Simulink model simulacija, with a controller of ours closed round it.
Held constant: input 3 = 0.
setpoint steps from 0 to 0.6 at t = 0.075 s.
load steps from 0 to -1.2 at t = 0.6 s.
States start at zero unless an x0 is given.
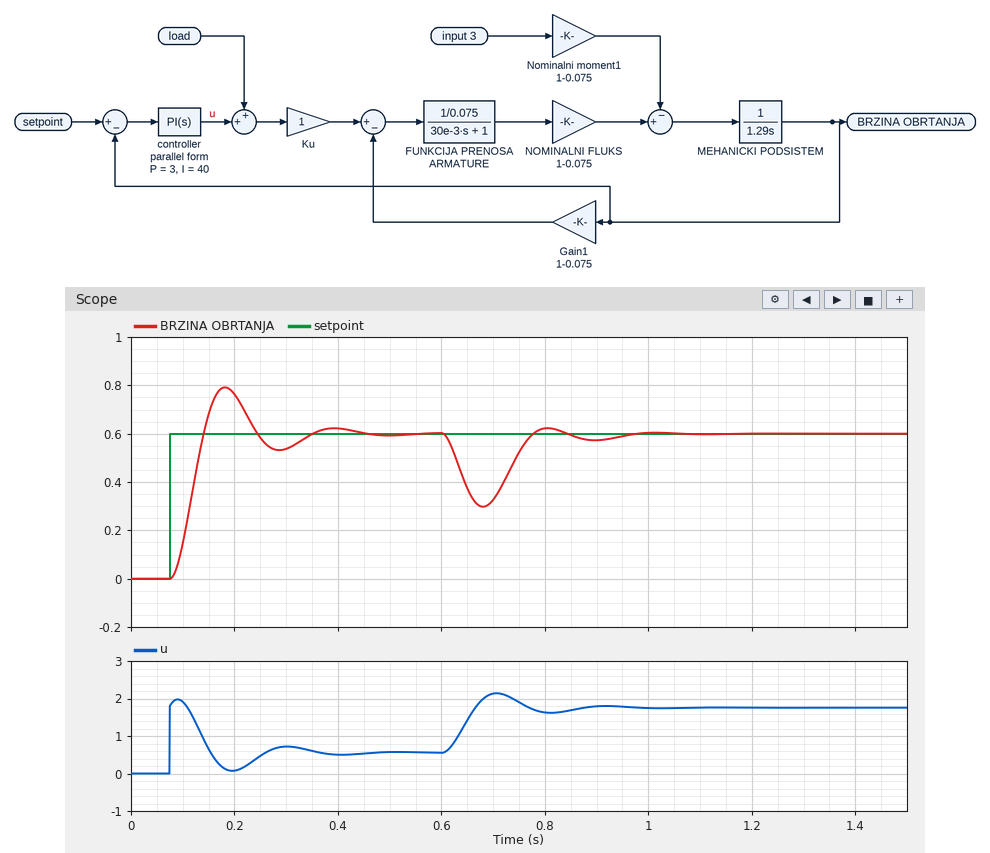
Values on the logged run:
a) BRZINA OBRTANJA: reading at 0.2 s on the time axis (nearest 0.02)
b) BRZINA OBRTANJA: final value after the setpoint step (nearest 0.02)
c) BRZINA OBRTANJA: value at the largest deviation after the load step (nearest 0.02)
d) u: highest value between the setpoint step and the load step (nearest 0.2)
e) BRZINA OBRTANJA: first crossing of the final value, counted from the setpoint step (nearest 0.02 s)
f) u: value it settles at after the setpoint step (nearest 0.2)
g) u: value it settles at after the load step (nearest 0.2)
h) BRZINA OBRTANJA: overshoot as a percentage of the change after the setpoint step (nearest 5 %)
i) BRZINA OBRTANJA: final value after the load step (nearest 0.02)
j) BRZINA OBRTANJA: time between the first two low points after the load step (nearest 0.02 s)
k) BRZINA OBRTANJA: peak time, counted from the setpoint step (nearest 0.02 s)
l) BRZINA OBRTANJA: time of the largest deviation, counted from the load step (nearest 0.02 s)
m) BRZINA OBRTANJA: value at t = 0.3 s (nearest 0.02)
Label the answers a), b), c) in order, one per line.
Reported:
a) 0.76
b) 0.60
c) 0.30
d) 2.0
e) 0.06 s
f) 0.6
g) 1.8
h) 30 %
i) 0.60
j) 0.22 s
k) 0.10 s
l) 0.08 s
m) 0.54
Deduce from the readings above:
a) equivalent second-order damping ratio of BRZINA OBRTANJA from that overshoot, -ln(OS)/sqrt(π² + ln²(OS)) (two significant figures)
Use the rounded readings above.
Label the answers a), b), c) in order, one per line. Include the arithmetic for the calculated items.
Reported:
a) ln(0.3) = -1.204; 1.204 / sqrt(9.870 + 1.450) = 0.36
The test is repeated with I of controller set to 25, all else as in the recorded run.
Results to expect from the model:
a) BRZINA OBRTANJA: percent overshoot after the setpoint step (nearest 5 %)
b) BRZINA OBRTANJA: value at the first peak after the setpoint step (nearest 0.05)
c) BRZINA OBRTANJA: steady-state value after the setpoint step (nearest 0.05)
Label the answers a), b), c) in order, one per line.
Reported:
a) 20 %
b) 0.70
c) 0.60
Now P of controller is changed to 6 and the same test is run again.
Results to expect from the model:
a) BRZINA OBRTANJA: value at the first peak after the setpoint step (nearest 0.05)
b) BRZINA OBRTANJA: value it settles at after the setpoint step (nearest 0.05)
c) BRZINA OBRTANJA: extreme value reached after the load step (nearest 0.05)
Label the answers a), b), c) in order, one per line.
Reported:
a) 0.80
b) 0.60
c) 0.40
